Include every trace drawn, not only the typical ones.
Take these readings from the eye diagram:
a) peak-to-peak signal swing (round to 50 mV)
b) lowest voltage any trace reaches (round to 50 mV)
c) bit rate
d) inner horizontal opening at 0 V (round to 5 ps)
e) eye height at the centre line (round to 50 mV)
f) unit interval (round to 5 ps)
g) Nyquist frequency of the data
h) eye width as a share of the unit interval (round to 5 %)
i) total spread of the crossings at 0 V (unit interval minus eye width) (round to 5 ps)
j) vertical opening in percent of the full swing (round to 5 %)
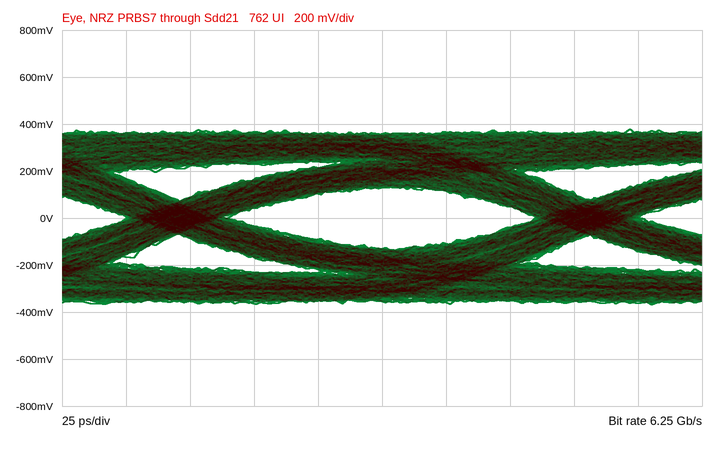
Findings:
750 mV
-350 mV
6.25 Gb/s
120 ps
250 mV
160 ps
3.125 GHz
75 %
40 ps
35 %
